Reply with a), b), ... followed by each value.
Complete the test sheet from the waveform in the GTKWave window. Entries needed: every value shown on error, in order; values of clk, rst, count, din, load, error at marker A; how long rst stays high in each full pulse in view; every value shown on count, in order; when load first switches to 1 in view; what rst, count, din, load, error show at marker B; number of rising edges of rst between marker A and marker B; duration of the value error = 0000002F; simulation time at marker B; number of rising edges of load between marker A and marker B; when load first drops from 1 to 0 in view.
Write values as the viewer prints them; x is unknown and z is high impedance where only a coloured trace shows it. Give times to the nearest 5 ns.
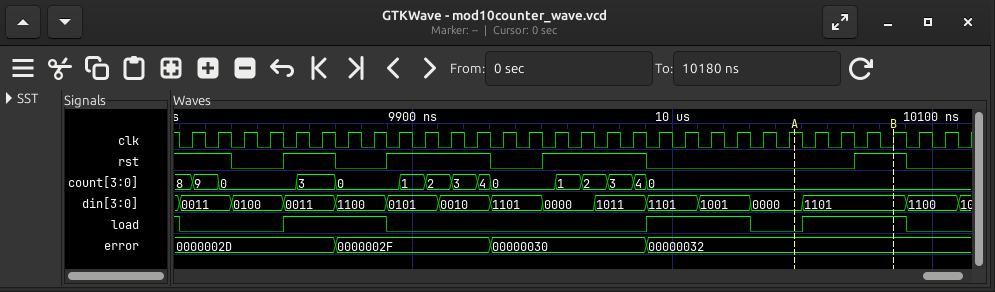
a) 0000002D, 0000002F, 00000030, 00000032
b) clk=1, rst=0, count=0, din=0000, load=0, error=00000032
c) 20 ns, 40 ns, 40 ns, 20 ns
d) 8, 9, 0, 3, 0, 1, 2, 3, 4, 0, 1, 2, 3, 4, 0
e) 9850 ns
f) rst=1, count=0, din=1101, load=1, error=00000032
g) 1
h) 60 ns
i) 10085 ns
j) 1
k) 9810 ns
